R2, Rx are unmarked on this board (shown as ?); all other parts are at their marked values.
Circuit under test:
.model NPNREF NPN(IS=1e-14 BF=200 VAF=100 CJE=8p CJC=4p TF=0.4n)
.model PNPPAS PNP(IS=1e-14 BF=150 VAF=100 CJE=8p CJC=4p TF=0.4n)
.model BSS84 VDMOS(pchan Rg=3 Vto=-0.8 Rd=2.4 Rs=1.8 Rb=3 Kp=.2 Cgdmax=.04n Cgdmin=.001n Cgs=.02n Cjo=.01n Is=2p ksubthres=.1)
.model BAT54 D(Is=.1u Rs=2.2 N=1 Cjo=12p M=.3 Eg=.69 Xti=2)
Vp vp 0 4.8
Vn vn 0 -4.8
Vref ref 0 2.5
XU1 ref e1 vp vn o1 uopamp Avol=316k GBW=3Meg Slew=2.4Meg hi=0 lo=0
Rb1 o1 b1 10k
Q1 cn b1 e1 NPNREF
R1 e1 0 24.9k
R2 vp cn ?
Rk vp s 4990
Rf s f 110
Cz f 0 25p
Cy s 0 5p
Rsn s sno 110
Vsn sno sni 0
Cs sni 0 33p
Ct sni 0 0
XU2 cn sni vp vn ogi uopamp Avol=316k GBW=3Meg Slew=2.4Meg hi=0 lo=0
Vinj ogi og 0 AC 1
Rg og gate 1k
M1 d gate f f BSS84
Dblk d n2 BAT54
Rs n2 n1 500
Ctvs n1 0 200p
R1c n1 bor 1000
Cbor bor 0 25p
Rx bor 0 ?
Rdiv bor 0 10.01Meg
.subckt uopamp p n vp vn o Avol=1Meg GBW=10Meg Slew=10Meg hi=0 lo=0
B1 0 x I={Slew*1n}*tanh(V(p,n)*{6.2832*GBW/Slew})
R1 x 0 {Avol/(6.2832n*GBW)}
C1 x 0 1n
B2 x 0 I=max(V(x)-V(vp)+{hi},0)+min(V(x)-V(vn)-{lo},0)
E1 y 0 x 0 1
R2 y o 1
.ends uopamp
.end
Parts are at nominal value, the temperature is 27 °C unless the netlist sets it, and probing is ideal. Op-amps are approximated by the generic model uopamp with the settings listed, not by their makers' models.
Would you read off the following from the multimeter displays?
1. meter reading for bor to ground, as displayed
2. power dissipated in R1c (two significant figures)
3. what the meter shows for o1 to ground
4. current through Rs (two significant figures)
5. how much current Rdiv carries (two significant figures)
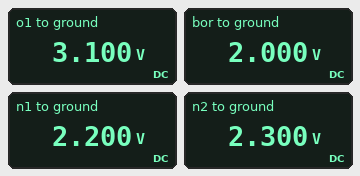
2.000 V
40 µW
3.100 V
200 µA
200 nA
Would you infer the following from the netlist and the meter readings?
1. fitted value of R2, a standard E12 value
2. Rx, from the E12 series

10 kΩ
10 kΩ
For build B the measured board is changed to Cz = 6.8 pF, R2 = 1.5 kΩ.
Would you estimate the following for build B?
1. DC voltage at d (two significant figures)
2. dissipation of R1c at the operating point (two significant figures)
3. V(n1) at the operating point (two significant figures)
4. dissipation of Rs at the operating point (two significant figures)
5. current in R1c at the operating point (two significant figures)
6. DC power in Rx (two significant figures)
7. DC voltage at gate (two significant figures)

490 mV
900 nW
330 mV
450 nW
30 µA
9.0 µW
4.0 V
